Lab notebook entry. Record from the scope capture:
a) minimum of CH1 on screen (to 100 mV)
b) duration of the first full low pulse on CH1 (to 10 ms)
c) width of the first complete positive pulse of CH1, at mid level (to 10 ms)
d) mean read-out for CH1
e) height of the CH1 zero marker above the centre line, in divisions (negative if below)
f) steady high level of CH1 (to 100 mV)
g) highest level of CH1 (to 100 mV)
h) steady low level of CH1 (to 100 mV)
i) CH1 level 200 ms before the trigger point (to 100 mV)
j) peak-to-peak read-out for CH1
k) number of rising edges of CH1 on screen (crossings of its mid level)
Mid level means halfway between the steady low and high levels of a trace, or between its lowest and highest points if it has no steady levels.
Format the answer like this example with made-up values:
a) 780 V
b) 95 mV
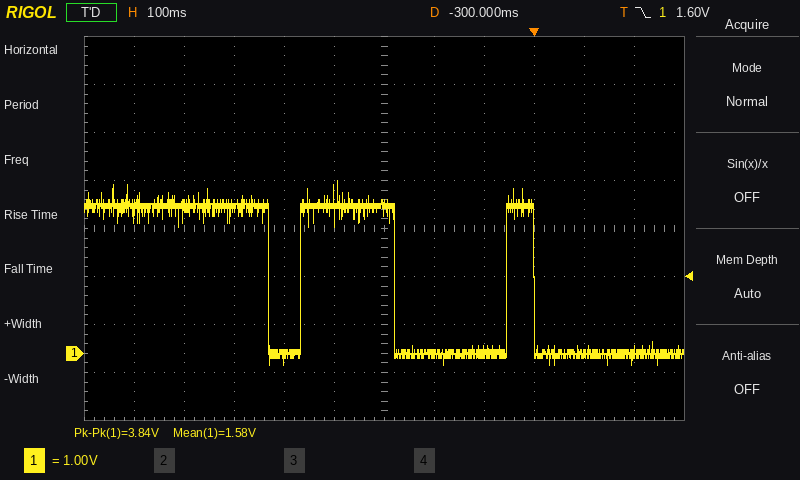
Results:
a) -200 mV
b) 60 ms
c) 190 ms
d) 1.58 V
e) -2.6 div
f) 3.1 V
g) 3.6 V
h) 0.0 V
i) 0.0 V
j) 3.84 V
k) 2
